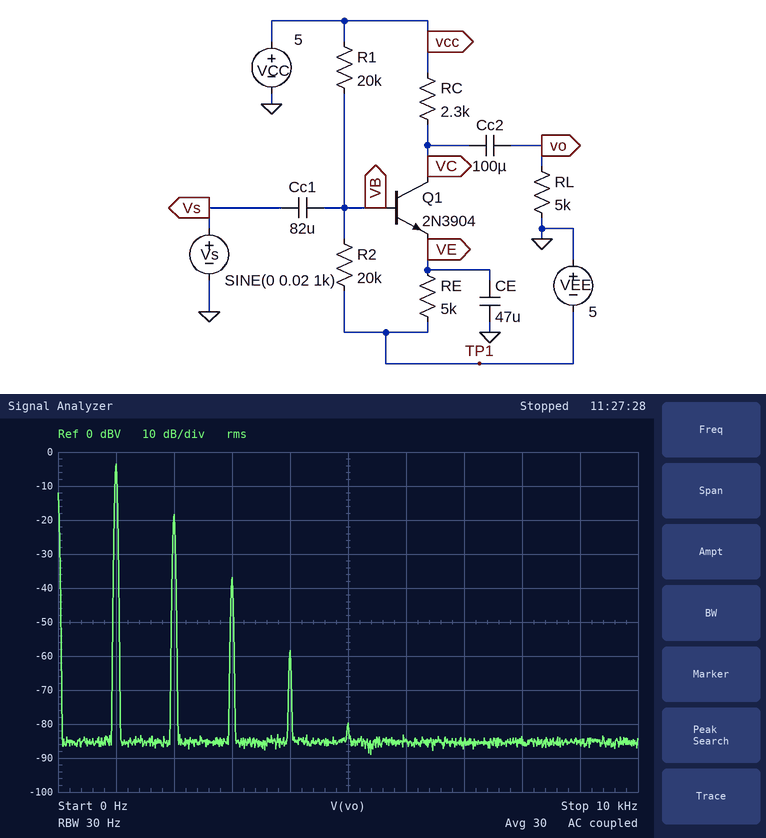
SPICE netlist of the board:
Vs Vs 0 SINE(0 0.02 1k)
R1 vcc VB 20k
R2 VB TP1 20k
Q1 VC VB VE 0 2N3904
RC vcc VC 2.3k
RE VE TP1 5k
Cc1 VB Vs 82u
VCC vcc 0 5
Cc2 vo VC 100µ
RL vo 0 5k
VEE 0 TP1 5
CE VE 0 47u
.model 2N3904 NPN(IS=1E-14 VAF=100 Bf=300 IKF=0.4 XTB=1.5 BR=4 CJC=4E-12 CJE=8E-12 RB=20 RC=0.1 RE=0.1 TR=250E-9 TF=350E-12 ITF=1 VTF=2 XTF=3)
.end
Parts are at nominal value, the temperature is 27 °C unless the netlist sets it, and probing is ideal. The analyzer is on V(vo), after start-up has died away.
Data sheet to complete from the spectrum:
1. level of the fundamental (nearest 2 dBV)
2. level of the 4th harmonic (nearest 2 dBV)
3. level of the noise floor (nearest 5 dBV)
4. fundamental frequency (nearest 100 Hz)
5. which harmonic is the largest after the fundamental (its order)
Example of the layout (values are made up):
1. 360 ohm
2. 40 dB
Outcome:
1. -4 dBV
2. -58 dBV
3. -85 dBV
4. 1.0 kHz
5. 2
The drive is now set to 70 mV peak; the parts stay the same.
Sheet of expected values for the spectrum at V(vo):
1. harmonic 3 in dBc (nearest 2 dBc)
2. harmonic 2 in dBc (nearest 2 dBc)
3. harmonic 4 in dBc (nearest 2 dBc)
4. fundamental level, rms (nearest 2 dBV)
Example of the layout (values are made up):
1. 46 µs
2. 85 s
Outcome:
1. -14 dBc
2. -6 dBc
3. -26 dBc
4. 4 dBV
